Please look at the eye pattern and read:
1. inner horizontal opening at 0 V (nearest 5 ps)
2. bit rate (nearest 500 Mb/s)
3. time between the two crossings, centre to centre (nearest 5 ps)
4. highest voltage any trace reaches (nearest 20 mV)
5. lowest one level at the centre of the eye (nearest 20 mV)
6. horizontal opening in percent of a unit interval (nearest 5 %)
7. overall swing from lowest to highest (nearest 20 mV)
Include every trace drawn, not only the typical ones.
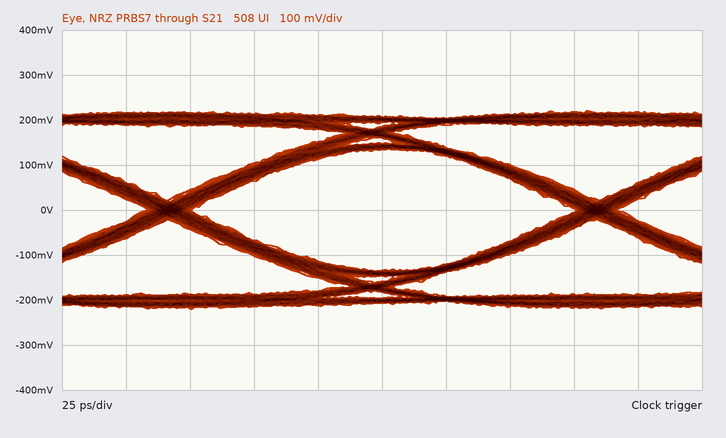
150 ps
6.0 Gb/s
165 ps
220 mV
140 mV
90 %
440 mV
